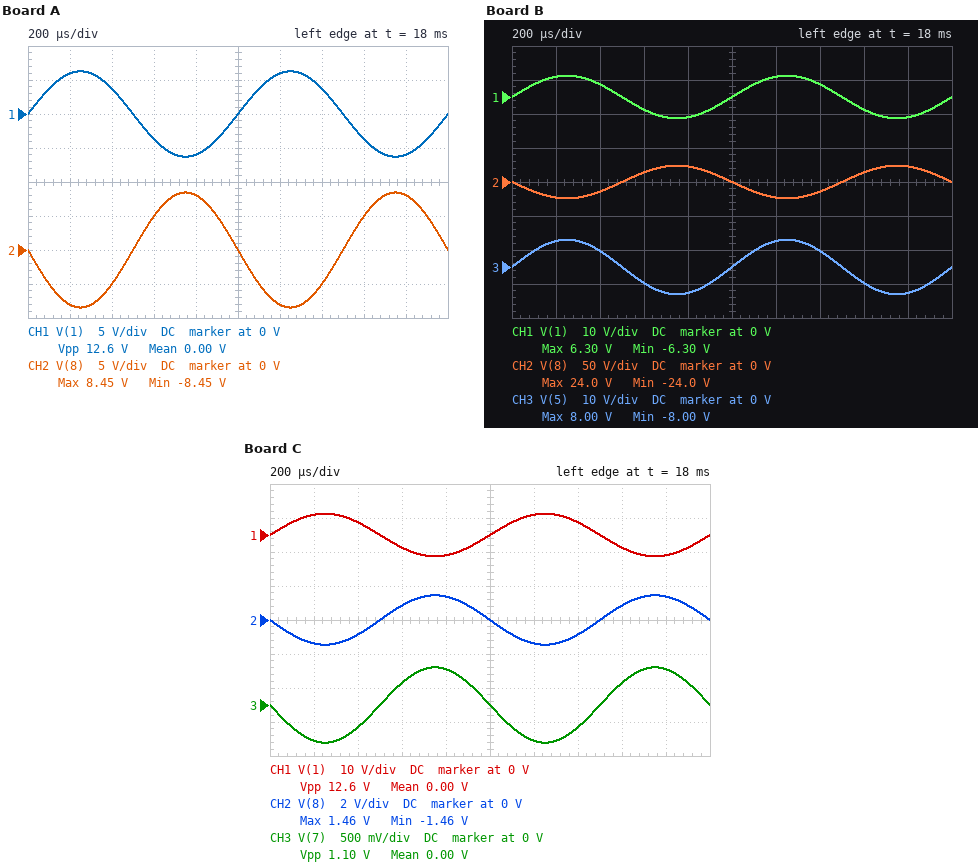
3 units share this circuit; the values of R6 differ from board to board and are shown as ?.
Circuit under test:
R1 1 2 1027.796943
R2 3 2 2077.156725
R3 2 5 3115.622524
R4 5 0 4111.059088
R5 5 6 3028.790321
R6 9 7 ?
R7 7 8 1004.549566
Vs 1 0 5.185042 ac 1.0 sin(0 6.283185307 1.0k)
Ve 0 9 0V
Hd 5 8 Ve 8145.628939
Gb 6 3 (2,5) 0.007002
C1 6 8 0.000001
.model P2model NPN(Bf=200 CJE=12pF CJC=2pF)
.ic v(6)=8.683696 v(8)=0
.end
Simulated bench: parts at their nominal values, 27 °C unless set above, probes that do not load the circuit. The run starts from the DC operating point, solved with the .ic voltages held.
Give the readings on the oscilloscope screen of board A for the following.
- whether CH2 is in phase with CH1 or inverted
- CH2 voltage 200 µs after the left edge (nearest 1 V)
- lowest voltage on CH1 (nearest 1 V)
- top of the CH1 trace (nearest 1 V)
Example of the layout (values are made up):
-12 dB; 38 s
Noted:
inverted; -8 V; -6 V; 6 V
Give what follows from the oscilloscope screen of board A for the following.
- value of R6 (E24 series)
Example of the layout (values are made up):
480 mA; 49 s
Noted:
3.6 kΩ
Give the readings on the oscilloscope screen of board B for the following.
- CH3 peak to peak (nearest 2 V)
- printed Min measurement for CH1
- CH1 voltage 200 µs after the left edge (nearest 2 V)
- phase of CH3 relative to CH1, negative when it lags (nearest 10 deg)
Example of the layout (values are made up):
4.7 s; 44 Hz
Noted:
16 V; -6.30 V; 6 V; 0 deg
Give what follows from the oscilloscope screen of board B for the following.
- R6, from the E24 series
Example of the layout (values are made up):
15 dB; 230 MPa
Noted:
5.1 kΩ
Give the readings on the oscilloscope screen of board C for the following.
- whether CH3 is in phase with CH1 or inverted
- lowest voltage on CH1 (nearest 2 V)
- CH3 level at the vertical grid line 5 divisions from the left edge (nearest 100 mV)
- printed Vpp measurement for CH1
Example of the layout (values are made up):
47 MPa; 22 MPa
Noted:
inverted; -6 V; 0 V; 12.6 V
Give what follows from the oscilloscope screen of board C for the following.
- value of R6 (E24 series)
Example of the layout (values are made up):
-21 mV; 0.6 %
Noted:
620 Ω
